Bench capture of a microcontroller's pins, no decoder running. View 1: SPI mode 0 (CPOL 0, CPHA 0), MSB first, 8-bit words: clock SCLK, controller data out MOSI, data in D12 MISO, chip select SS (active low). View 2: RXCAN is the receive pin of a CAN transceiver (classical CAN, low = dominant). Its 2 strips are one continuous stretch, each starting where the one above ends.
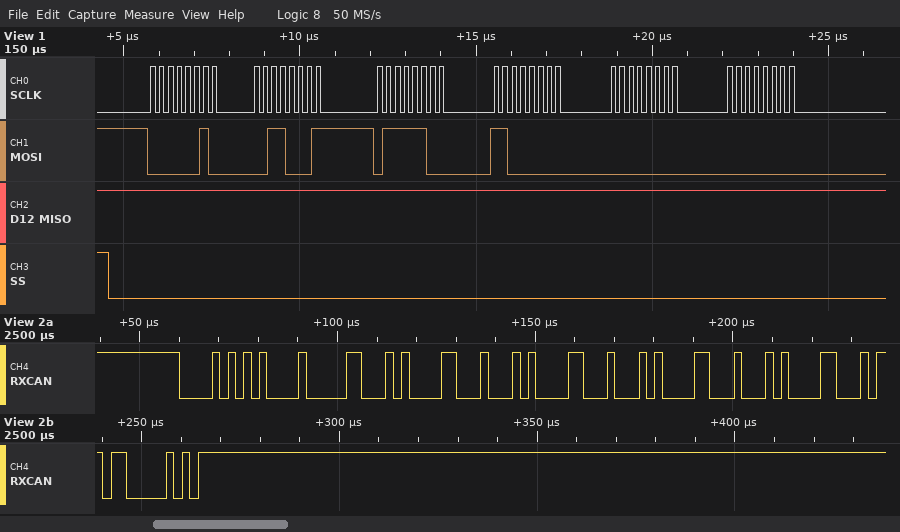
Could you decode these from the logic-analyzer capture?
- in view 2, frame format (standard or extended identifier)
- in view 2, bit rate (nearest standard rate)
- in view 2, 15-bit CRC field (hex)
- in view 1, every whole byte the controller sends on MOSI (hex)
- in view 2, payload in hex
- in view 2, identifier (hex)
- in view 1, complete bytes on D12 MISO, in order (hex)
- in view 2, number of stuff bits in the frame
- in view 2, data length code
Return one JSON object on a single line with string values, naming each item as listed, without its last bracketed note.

{"in view 2, frame format": "standard", "in view 2, bit rate": "500 kbit/s", "in view 2, 15-bit CRC field": "0x16C0", "in view 1, every whole byte the controller sends on MOSI": "0x02 0x31 0x7C 0xC0 0x00 0x00", "in view 2, payload in hex": "22 86 22 86 22 86 22 86", "in view 2, identifier": "0x0AA", "in view 1, complete bytes on D12 MISO, in order": "0xFF 0xFF 0xFF 0xFF 0xFF 0xFF", "in view 2, number of stuff bits in the frame": "2", "in view 2, data length code": "8"}
